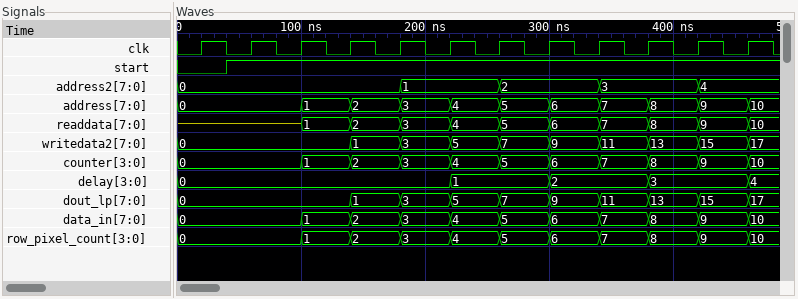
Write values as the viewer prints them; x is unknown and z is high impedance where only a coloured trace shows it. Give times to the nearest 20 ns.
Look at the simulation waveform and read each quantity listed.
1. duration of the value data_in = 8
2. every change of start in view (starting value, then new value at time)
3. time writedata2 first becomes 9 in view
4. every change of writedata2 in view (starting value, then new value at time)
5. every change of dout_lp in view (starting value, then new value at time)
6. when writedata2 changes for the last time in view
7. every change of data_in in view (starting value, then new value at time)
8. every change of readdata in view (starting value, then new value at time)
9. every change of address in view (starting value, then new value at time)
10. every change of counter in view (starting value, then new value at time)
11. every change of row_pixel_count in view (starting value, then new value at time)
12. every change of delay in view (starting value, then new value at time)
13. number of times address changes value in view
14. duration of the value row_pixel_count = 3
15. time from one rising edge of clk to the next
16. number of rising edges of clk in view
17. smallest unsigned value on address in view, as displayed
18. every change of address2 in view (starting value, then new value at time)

40 ns
0, 1 at 40 ns
300 ns
0, 1 at 140 ns, 3 at 180 ns, 5 at 220 ns, 7 at 260 ns, 9 at 300 ns, 11 at 340 ns, 13 at 380 ns, 15 at 420 ns, 17 at 460 ns
0, 1 at 140 ns, 3 at 180 ns, 5 at 220 ns, 7 at 260 ns, 9 at 300 ns, 11 at 340 ns, 13 at 380 ns, 15 at 420 ns, 17 at 460 ns
460 ns
0, 1 at 100 ns, 2 at 140 ns, 3 at 180 ns, 4 at 220 ns, 5 at 260 ns, 6 at 300 ns, 7 at 340 ns, 8 at 380 ns, 9 at 420 ns, 10 at 460 ns
z, 1 at 100 ns, 2 at 140 ns, 3 at 180 ns, 4 at 220 ns, 5 at 260 ns, 6 at 300 ns, 7 at 340 ns, 8 at 380 ns, 9 at 420 ns, 10 at 460 ns
0, 1 at 100 ns, 2 at 140 ns, 3 at 180 ns, 4 at 220 ns, 5 at 260 ns, 6 at 300 ns, 7 at 340 ns, 8 at 380 ns, 9 at 420 ns, 10 at 460 ns
0, 1 at 100 ns, 2 at 140 ns, 3 at 180 ns, 4 at 220 ns, 5 at 260 ns, 6 at 300 ns, 7 at 340 ns, 8 at 380 ns, 9 at 420 ns, 10 at 460 ns
0, 1 at 100 ns, 2 at 140 ns, 3 at 180 ns, 4 at 220 ns, 5 at 260 ns, 6 at 300 ns, 7 at 340 ns, 8 at 380 ns, 9 at 420 ns, 10 at 460 ns
0, 1 at 220 ns, 2 at 300 ns, 3 at 380 ns, 4 at 460 ns
10
40 ns
40 ns
12
0
0, 1 at 180 ns, 2 at 260 ns, 3 at 340 ns, 4 at 420 ns
